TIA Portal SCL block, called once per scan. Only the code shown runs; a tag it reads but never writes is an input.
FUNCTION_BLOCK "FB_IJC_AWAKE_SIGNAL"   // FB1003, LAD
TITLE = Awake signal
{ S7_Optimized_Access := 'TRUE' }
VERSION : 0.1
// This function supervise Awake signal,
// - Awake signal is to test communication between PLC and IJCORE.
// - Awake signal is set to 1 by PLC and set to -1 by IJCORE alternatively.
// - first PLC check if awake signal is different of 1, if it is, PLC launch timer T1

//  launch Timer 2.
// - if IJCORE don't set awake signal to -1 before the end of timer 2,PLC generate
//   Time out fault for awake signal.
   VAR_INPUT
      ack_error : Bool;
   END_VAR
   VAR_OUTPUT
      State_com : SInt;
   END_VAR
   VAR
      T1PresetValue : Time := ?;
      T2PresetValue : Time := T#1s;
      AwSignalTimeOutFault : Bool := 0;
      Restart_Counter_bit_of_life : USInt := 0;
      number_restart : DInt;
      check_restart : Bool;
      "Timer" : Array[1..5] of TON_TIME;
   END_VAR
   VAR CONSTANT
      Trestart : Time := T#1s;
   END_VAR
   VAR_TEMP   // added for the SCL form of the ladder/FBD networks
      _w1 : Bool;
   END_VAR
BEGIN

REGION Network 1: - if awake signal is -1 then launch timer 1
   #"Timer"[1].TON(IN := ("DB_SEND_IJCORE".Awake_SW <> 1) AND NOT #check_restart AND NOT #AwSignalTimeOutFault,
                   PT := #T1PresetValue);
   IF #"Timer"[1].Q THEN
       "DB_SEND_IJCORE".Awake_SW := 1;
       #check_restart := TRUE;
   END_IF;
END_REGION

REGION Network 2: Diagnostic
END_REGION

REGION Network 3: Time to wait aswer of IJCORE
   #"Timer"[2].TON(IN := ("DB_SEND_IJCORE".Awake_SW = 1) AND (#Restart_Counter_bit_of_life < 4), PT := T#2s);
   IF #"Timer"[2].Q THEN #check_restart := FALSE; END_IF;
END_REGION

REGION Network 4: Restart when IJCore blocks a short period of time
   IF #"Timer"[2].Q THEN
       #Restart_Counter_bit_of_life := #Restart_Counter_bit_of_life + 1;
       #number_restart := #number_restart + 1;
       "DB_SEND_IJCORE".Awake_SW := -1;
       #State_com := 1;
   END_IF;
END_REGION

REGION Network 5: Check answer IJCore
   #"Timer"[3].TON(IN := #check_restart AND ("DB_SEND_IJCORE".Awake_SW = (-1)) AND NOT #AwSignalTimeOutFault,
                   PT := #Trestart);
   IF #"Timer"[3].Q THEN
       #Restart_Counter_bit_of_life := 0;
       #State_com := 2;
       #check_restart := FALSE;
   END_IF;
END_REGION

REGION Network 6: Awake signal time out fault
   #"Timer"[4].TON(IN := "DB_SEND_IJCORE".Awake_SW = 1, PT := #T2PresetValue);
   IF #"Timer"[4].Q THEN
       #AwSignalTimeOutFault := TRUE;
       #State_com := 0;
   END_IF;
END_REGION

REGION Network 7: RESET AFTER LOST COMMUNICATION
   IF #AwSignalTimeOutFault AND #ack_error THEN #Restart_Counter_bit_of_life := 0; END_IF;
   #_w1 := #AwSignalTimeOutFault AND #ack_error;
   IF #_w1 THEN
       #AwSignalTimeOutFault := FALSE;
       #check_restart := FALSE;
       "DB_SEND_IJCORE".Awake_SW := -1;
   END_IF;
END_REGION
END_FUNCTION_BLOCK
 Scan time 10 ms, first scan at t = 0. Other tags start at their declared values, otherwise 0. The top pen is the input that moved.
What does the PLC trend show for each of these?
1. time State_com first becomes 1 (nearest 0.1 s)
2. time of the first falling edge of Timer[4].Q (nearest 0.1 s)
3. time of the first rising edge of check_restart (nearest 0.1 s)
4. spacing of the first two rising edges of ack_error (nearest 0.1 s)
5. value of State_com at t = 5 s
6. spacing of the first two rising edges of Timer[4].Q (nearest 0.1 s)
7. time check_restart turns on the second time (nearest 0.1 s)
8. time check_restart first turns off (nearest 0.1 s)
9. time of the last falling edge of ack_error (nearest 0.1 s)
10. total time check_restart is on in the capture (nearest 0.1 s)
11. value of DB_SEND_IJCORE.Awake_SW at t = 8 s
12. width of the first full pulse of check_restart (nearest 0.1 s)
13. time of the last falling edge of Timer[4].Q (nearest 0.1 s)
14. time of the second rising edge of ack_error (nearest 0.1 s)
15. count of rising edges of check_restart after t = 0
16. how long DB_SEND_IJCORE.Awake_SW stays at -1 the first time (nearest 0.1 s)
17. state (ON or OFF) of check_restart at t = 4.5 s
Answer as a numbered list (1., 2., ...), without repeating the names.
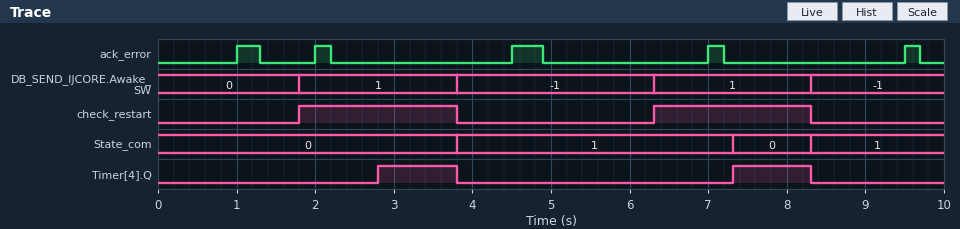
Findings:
1. 3.8 s
2. 3.8 s
3. 1.8 s
4. 1.0 s
5. 1
6. 4.5 s
7. 6.3 s
8. 3.8 s
9. 9.7 s
10. 4.0 s
11. 1
12. 2.0 s
13. 8.3 s
14. 2.0 s
15. 2
16. 2.5 s
17. OFF
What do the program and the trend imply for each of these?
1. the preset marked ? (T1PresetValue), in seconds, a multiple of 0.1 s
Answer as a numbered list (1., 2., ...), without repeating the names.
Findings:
1. 1.8 s
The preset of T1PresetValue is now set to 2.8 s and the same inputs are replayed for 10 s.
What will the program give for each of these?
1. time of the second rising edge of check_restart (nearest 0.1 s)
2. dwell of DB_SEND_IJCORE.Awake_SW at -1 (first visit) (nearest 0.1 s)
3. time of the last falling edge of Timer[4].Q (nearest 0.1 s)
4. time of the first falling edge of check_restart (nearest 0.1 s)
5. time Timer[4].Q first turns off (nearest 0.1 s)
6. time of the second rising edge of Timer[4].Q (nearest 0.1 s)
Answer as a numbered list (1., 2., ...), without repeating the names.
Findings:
1. 7.3 s
2. 2.8 s
3. 9.3 s
4. 4.5 s
5. 4.5 s
6. 8.3 s
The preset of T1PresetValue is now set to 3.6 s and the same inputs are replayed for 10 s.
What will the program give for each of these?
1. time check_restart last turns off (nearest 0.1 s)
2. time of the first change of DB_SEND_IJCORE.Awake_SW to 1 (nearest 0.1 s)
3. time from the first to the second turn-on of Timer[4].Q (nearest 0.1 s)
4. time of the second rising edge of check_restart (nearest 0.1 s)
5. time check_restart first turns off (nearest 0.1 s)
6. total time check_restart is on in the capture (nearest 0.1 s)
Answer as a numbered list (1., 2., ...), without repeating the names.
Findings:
1. 9.5 s
2. 3.6 s
3. 4.6 s
4. 8.2 s
5. 4.6 s
6. 2.3 s
